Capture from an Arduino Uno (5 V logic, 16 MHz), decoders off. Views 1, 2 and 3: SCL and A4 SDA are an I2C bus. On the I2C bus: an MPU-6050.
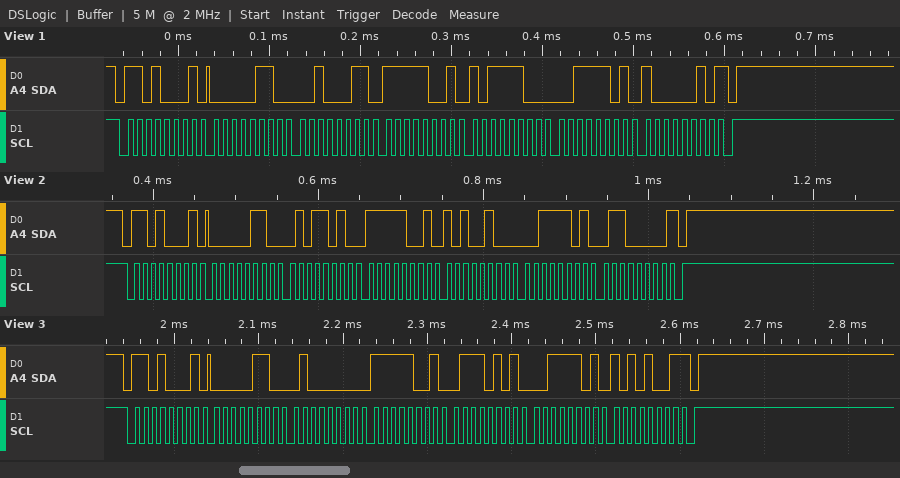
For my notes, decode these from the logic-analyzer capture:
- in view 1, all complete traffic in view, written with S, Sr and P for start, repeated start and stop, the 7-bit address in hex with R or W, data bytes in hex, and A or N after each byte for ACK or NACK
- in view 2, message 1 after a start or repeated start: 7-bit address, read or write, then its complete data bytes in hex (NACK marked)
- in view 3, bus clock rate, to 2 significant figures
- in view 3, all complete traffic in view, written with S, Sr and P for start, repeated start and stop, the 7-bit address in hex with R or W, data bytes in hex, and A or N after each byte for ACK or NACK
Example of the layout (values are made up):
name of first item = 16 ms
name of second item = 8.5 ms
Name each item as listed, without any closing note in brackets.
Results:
in view 1, all complete traffic in view, written with S, Sr and P for start, repeated start and stop, the 7-bit address in hex with R or W, data bytes in hex, and A or N after each byte for ACK or NACK = S 68R A 06 A 23 A F9 A BC A 3D A 82 N P
in view 2, message 1 after a start or repeated start: 7-bit address, read or write, then its complete data bytes in hex = 0x68 read: 06 5A F9 A4 3D 60 NACK
in view 3, bus clock rate, to 2 significant figures = 100 kHz
in view 3, all complete traffic in view, written with S, Sr and P for start, repeated start and stop, the 7-bit address in hex with R or W, data bytes in hex, and A or N after each byte for ACK or NACK = S 68R A 06 A 40 A F9 A 75 A 3D A A9 N P
